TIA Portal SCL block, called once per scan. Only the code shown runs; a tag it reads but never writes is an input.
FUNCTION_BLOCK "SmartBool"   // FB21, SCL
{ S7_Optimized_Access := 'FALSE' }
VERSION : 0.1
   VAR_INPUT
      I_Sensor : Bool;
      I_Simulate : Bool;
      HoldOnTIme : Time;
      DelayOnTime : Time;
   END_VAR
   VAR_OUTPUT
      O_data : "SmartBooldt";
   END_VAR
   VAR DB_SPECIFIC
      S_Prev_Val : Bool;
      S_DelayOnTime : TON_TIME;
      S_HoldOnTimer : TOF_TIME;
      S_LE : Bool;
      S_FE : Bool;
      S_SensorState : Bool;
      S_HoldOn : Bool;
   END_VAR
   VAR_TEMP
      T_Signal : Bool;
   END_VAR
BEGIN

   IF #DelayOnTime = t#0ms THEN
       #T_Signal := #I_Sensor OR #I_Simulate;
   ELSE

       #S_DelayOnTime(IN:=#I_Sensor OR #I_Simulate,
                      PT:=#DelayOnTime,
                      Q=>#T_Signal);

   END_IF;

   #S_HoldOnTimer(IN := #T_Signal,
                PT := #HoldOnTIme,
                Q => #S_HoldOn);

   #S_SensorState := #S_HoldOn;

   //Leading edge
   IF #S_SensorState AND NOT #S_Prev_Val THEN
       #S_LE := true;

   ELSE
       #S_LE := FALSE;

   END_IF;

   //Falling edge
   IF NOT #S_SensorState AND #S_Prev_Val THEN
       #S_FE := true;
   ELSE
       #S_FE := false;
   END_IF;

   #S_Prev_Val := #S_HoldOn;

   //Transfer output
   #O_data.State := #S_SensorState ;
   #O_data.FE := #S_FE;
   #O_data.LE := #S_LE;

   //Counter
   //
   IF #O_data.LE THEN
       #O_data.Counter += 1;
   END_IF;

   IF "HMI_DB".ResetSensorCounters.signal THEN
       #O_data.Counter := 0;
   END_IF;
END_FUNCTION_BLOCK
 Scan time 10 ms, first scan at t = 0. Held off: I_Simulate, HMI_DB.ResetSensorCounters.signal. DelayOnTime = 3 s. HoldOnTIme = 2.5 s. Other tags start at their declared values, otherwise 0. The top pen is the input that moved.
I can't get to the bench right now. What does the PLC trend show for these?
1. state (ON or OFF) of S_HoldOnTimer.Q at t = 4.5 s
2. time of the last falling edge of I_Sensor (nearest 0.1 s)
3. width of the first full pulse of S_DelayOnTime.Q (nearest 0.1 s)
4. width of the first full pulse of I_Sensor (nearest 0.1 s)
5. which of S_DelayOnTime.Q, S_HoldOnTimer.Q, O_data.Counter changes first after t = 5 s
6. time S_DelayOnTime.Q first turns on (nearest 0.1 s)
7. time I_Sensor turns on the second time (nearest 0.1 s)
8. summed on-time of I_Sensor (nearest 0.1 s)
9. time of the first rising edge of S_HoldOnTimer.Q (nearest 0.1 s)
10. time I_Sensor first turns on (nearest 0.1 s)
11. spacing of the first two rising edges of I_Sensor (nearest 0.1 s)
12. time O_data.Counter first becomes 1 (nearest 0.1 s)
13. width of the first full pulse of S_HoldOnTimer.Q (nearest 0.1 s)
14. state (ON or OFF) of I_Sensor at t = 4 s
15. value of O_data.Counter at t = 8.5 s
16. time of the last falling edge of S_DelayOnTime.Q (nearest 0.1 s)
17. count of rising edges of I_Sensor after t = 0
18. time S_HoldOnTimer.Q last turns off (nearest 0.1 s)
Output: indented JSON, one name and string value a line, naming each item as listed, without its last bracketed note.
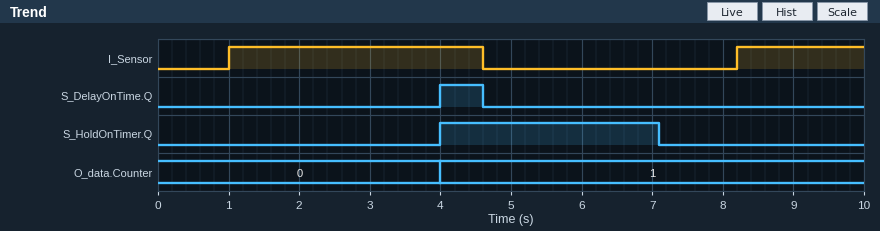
{
  "state (ON or OFF) of S_HoldOnTimer.Q at t = 4.5 s": "ON",
  "time of the last falling edge of I_Sensor": "4.6 s",
  "width of the first full pulse of S_DelayOnTime.Q": "0.6 s",
  "width of the first full pulse of I_Sensor": "3.6 s",
  "which of S_DelayOnTime.Q, S_HoldOnTimer.Q, O_data.Counter changes first after t = 5 s": "S_HoldOnTimer.Q",
  "time S_DelayOnTime.Q first turns on": "4.0 s",
  "time I_Sensor turns on the second time": "8.2 s",
  "summed on-time of I_Sensor": "5.4 s",
  "time of the first rising edge of S_HoldOnTimer.Q": "4.0 s",
  "time I_Sensor first turns on": "1.0 s",
  "spacing of the first two rising edges of I_Sensor": "7.2 s",
  "time O_data.Counter first becomes 1": "4.0 s",
  "width of the first full pulse of S_HoldOnTimer.Q": "3.1 s",
  "state (ON or OFF) of I_Sensor at t = 4 s": "ON",
  "value of O_data.Counter at t = 8.5 s": "1",
  "time of the last falling edge of S_DelayOnTime.Q": "4.6 s",
  "count of rising edges of I_Sensor after t = 0": "2",
  "time S_HoldOnTimer.Q last turns off": "7.1 s"
}
